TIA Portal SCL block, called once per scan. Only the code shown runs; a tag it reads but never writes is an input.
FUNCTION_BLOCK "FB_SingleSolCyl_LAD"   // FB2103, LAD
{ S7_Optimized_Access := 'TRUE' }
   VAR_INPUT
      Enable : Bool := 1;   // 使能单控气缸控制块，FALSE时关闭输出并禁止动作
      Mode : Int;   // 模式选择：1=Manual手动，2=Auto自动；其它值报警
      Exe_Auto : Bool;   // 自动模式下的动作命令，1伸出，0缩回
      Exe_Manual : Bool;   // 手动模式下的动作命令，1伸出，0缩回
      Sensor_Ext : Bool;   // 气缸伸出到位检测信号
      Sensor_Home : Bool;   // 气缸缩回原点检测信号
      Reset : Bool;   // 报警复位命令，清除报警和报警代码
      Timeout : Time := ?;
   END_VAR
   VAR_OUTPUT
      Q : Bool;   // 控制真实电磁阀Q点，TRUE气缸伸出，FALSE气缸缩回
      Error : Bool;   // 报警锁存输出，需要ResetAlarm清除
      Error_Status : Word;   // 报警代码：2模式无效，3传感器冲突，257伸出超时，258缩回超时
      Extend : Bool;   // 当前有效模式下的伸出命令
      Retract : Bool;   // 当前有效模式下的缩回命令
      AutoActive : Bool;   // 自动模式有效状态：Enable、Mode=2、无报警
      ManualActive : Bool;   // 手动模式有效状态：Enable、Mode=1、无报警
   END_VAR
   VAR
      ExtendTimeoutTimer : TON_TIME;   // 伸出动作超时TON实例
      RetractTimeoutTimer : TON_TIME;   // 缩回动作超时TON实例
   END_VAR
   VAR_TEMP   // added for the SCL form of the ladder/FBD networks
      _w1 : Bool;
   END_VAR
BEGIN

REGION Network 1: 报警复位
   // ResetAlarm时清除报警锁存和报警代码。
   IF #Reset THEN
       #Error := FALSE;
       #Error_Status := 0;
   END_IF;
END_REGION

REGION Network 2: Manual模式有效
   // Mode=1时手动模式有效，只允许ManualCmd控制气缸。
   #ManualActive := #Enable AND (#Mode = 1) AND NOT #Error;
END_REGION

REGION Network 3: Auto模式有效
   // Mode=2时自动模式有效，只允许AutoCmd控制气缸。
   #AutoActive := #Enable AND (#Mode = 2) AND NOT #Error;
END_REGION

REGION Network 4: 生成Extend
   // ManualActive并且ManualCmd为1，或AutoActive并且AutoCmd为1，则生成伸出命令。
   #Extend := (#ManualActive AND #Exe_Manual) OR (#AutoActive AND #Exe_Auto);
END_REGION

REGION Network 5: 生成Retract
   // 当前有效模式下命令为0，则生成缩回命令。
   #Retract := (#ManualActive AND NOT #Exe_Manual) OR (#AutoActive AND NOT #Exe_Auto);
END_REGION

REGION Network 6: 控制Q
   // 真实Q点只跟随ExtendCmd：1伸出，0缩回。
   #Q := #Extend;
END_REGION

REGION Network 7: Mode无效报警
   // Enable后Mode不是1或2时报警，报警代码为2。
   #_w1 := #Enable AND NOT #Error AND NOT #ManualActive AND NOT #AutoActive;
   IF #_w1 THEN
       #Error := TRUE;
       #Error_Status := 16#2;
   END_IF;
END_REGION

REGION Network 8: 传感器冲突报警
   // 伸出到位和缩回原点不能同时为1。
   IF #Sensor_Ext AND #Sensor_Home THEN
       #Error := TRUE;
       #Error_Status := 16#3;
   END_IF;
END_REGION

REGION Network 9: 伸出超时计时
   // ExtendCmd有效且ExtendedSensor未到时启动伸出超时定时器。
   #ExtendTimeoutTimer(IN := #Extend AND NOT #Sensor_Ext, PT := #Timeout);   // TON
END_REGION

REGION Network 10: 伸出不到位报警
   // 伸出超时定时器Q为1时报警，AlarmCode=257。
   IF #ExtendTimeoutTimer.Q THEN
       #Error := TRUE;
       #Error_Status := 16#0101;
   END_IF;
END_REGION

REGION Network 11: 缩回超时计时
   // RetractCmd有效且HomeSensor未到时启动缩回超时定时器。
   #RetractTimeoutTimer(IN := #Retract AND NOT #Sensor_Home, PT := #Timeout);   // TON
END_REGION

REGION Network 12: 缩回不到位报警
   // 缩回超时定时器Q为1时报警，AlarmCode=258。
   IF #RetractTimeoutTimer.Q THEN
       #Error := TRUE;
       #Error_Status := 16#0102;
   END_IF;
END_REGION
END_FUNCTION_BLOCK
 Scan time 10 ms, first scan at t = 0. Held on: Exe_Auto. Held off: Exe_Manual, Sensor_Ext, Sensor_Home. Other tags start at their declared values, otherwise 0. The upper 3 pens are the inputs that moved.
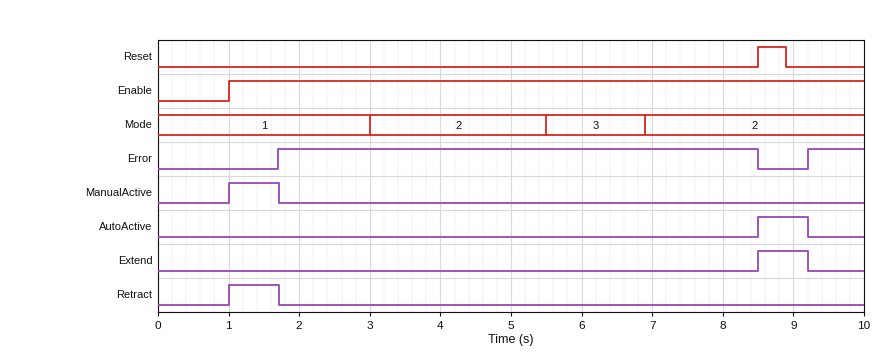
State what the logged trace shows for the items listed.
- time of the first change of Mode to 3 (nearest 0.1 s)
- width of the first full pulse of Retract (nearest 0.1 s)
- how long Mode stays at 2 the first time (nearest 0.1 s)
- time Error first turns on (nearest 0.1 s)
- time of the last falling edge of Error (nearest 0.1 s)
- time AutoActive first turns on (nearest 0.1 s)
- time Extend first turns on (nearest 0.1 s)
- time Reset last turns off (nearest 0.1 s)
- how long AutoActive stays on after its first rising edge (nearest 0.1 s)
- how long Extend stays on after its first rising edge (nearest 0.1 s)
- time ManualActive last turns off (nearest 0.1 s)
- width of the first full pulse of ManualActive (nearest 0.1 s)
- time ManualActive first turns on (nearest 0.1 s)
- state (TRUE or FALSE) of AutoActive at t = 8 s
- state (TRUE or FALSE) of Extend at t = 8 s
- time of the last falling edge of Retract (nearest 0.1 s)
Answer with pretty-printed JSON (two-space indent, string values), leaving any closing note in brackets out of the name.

{
  "time of the first change of Mode to 3": "5.5 s",
  "width of the first full pulse of Retract": "0.7 s",
  "how long Mode stays at 2 the first time": "2.5 s",
  "time Error first turns on": "1.7 s",
  "time of the last falling edge of Error": "8.5 s",
  "time AutoActive first turns on": "8.5 s",
  "time Extend first turns on": "8.5 s",
  "time Reset last turns off": "8.9 s",
  "how long AutoActive stays on after its first rising edge": "0.7 s",
  "how long Extend stays on after its first rising edge": "0.7 s",
  "time ManualActive last turns off": "1.7 s",
  "width of the first full pulse of ManualActive": "0.7 s",
  "time ManualActive first turns on": "1.0 s",
  "state (TRUE or FALSE) of AutoActive at t = 8 s": "FALSE",
  "state (TRUE or FALSE) of Extend at t = 8 s": "FALSE",
  "time of the last falling edge of Retract": "1.7 s"
}
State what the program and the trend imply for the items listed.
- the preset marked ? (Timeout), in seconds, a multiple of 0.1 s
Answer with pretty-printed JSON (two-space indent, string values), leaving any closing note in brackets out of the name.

{
  "the preset marked ? (Timeout), in seconds, a multiple of 0.1 s": "0.7 s"
}
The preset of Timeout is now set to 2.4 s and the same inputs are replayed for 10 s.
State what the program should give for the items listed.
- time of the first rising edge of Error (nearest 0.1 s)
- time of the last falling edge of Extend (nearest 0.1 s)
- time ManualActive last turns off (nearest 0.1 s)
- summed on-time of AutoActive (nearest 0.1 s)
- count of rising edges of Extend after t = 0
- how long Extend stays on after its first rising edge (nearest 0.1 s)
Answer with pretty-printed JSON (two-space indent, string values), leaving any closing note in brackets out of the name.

{
  "time of the first rising edge of Error": "5.4 s",
  "time of the last falling edge of Extend": "5.4 s",
  "time ManualActive last turns off": "3.0 s",
  "summed on-time of AutoActive": "3.9 s",
  "count of rising edges of Extend after t = 0": "2",
  "how long Extend stays on after its first rising edge": "2.4 s"
}
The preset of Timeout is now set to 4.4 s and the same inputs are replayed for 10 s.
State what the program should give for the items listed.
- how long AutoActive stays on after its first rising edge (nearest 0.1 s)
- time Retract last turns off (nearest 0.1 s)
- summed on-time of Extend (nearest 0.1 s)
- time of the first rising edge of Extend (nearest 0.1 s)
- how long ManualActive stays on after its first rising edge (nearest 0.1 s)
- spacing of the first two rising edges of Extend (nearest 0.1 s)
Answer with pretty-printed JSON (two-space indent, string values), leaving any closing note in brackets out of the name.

{
  "how long AutoActive stays on after its first rising edge": "2.5 s",
  "time Retract last turns off": "3.0 s",
  "summed on-time of Extend": "4.0 s",
  "time of the first rising edge of Extend": "3.0 s",
  "how long ManualActive stays on after its first rising edge": "2.0 s",
  "spacing of the first two rising edges of Extend": "5.5 s"
}
